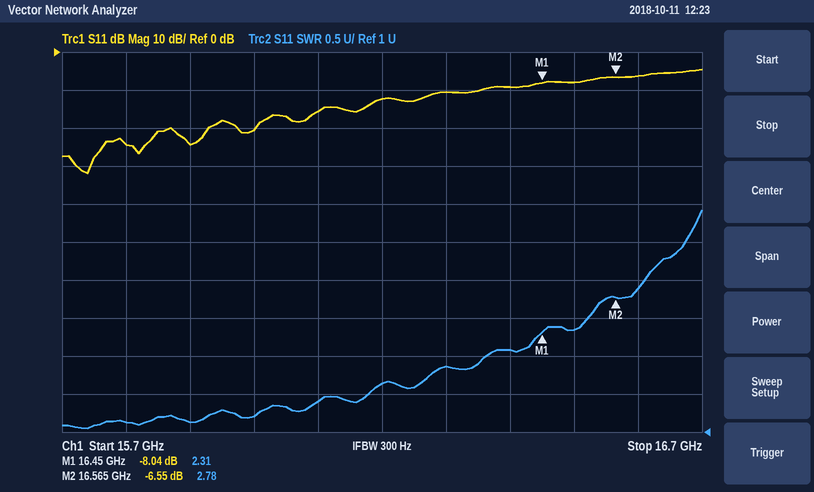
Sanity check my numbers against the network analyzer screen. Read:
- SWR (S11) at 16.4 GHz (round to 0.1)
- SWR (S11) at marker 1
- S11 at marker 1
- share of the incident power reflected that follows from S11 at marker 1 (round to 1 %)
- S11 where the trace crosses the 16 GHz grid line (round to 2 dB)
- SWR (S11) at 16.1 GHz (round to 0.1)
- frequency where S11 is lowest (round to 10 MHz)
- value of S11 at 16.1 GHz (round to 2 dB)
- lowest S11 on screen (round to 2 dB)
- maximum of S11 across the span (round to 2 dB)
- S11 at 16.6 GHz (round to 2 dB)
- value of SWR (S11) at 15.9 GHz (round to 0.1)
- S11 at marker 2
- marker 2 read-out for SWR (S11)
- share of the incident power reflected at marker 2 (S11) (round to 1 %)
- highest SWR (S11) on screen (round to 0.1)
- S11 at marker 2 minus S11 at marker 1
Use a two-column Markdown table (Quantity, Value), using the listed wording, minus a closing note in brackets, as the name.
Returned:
| Quantity | Value |
|---|---|
| SWR (S11) at 16.4 GHz | 2.1 |
| SWR (S11) at marker 1 | 2.31 |
| S11 at marker 1 | -8.04 dB |
| share of the incident power reflected that follows from S11 at marker 1 | 16 % |
| S11 where the trace crosses the 16 GHz grid line | -20 dB |
| SWR (S11) at 16.1 GHz | 1.4 |
| frequency where S11 is lowest | 15.74 GHz |
| value of S11 at 16.1 GHz | -16 dB |
| lowest S11 on screen | -32 dB |
| maximum of S11 across the span | -4 dB |
| S11 at 16.6 GHz | -6 dB |
| value of SWR (S11) at 15.9 GHz | 1.1 |
| S11 at marker 2 | -6.55 dB |
| marker 2 read-out for SWR | 2.78 |
| share of the incident power reflected at marker 2 (S11) | 22 % |
| highest SWR (S11) on screen | 3.9 |
| S11 at marker 2 minus S11 at marker 1 | 1.49 dB |
